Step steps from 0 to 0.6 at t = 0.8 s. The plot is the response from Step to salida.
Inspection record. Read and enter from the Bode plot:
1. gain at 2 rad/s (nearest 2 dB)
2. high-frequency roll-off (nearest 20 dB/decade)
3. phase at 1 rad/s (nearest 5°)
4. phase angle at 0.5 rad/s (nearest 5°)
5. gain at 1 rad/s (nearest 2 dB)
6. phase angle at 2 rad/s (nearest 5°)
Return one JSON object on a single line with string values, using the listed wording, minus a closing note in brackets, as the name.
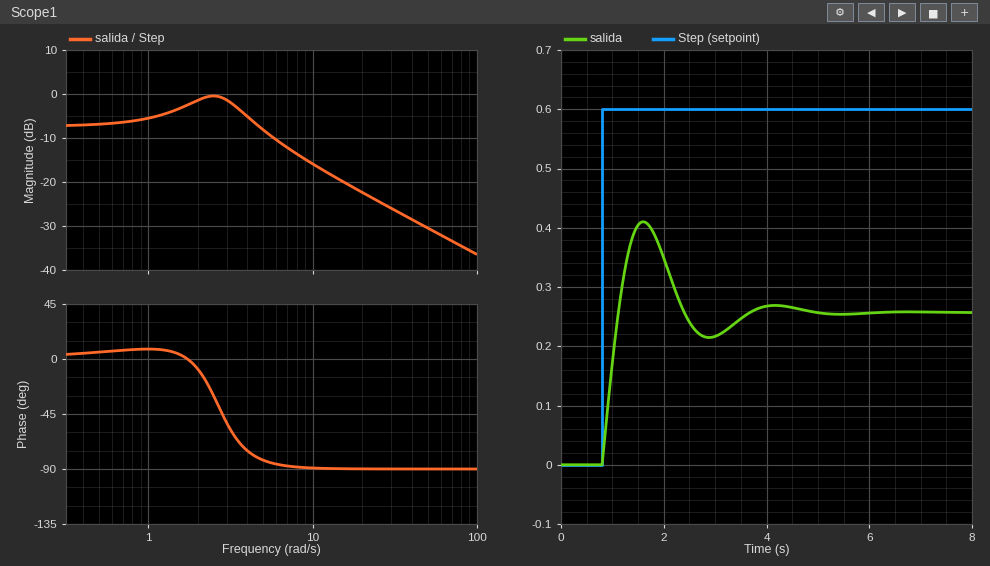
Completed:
{"gain at 2 rad/s": "-2 dB", "high-frequency roll-off": "-20 dB/decade", "phase at 1 rad/s": "10°", "phase angle at 0.5 rad/s": "5°", "gain at 1 rad/s": "-6 dB", "phase angle at 2 rad/s": "-10°"}
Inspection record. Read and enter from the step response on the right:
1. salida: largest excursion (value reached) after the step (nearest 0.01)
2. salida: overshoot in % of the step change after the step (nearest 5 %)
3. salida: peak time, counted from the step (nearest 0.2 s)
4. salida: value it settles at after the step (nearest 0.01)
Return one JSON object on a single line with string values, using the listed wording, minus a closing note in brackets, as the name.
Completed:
{"salida: largest excursion (value reached) after the step": "0.41", "salida: overshoot in % of the step change after the step": "60 %", "salida: peak time, counted from the step": "0.8 s", "salida: value it settles at after the step": "0.26"}
